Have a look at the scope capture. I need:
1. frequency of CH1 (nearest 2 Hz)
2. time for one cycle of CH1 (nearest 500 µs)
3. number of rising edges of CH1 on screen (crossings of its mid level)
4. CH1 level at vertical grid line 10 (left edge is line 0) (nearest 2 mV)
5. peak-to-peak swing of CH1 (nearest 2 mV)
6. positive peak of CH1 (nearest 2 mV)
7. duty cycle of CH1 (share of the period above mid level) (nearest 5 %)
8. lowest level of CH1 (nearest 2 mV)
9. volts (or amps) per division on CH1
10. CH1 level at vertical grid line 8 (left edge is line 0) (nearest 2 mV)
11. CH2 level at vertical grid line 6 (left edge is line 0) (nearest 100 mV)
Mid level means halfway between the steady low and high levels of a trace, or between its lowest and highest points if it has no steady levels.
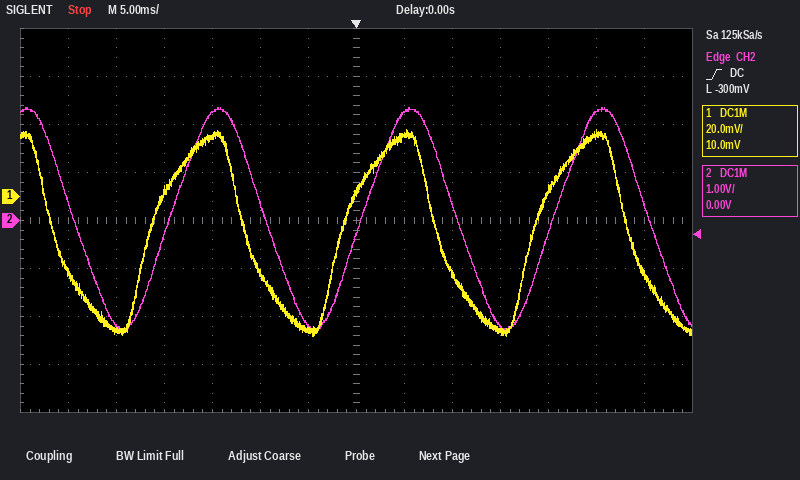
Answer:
50 Hz
20.0 ms
3
-56 mV
86 mV
28 mV
50 %
-58 mV
20 mV
26 mV
-2.2 V
